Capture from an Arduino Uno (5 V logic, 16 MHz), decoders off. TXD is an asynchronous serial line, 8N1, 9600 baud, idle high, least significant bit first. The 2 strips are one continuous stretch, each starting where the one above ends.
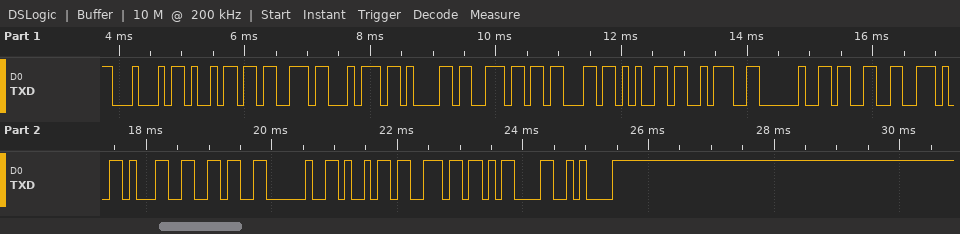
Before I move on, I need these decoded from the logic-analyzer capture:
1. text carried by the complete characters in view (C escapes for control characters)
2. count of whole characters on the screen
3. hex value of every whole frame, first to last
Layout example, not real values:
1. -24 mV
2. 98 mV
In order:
1. "Distance: 3.16 in\r\n"
2. 19
3. 44 69 73 74 61 6E 63 65 3A 20 33 2E 31 36 20 69 6E 0D 0A
